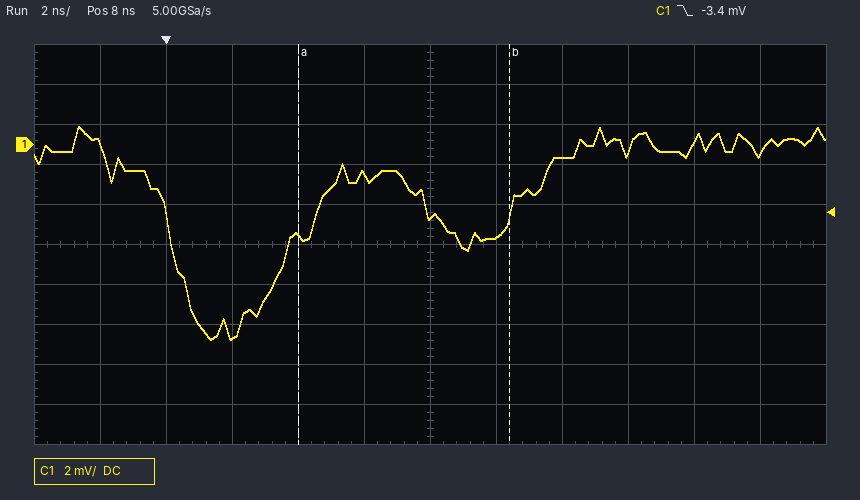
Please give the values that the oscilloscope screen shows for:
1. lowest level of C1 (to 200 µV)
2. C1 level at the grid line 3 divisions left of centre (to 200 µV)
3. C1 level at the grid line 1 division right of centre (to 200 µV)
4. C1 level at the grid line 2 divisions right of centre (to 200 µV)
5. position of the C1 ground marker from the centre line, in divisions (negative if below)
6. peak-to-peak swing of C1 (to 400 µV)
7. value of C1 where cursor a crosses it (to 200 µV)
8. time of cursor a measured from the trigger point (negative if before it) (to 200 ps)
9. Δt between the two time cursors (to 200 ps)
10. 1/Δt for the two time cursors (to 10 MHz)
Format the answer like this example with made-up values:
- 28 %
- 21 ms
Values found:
- -9.8 mV
- -9.6 mV
- -4.6 mV
- -600 µV
- +2.5 div
- 10.8 mV
- -4.6 mV
- +4.0 ns
- 6.4 ns
- 160 MHz
